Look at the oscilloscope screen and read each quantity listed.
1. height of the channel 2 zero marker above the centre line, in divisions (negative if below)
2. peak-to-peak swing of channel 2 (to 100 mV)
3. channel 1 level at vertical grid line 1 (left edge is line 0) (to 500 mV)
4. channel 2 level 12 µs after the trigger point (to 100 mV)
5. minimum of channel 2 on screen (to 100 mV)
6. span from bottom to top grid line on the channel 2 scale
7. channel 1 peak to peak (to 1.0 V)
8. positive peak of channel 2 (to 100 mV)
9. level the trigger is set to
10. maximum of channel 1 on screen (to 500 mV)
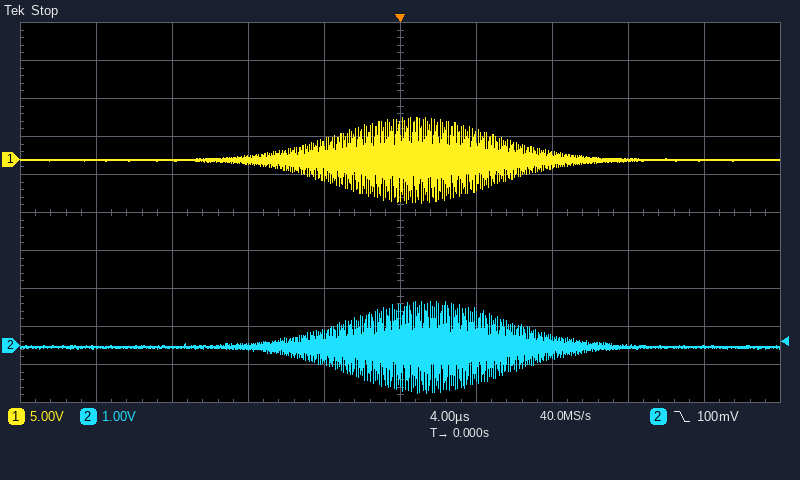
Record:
-3.5 div
2.4 V
0.0 V
0.0 V
-1.2 V
10 V
11.0 V
1.2 V
100 mV
5.5 V
